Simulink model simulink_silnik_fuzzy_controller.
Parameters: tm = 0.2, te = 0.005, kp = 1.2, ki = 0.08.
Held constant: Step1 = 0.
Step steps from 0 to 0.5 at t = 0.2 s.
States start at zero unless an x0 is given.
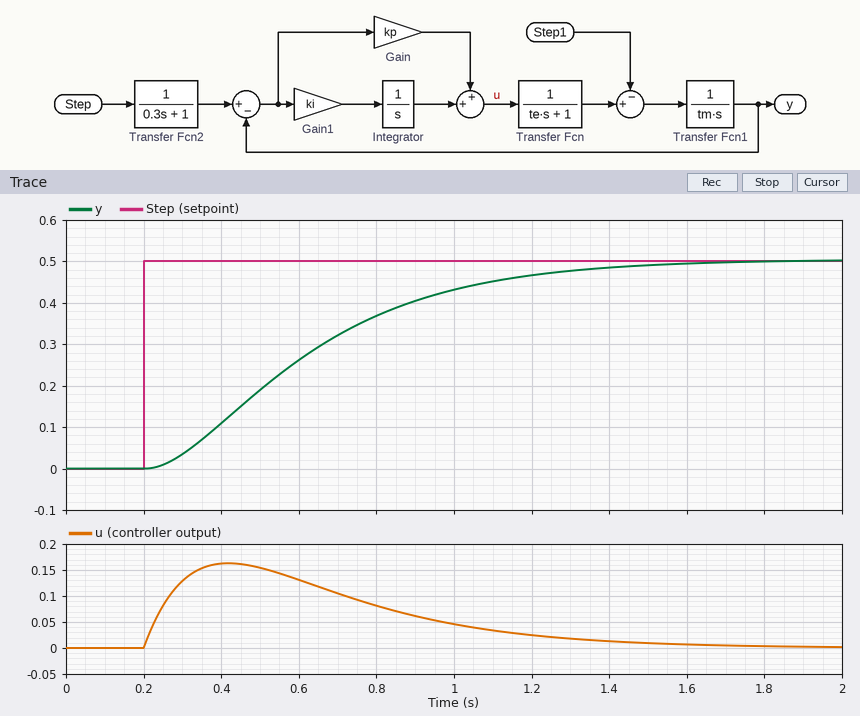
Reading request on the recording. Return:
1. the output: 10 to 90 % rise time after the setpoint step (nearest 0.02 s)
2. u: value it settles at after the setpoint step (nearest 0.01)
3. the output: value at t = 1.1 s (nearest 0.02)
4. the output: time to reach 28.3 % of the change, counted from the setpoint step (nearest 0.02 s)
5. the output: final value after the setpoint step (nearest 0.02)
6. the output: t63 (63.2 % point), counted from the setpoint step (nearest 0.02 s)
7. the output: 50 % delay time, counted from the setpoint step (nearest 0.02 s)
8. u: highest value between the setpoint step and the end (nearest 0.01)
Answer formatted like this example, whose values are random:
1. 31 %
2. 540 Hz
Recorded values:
1. 0.78 s
2. 0.00
3. 0.46
4. 0.24 s
5. 0.50
6. 0.50 s
7. 0.38 s
8. 0.16
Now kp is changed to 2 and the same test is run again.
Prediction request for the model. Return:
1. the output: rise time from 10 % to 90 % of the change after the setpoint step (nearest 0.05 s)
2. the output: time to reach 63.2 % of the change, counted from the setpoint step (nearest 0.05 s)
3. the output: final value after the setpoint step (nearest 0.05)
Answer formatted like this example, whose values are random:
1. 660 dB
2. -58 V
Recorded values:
1. 0.70 s
2. 0.40 s
3. 0.50
